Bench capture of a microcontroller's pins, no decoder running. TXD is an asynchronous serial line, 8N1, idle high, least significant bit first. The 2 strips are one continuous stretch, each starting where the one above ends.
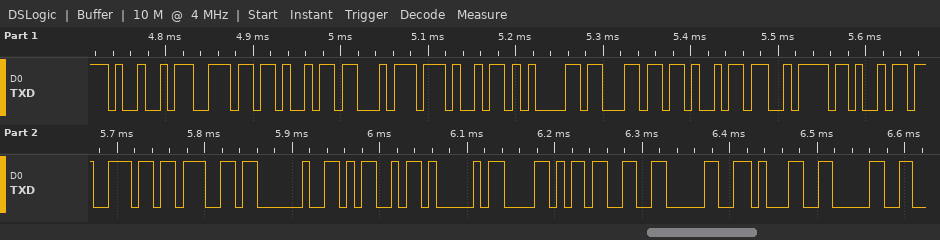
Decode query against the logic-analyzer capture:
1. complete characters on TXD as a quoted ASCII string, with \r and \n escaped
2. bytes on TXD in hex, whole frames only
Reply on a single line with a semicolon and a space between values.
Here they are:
"Initializing MAX3010"; 49 6E 69 74 69 61 6C 69 7A 69 6E 67 20 4D 41 58 33 30 31 30
